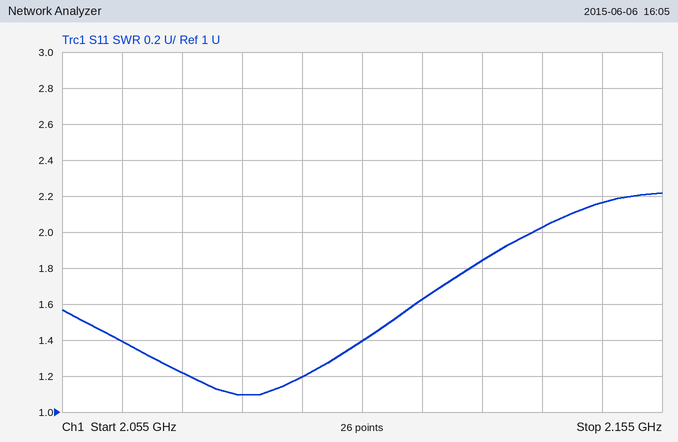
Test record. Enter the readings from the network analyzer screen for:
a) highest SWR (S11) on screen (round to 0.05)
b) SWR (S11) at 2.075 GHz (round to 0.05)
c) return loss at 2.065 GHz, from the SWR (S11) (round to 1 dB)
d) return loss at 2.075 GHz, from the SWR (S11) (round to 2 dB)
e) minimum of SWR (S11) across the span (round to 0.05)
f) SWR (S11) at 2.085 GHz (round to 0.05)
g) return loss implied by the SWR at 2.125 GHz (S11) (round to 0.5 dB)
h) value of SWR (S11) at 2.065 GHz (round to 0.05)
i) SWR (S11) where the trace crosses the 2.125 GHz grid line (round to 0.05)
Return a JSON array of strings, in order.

["2.20", "1.20", "16 dB", "20 dB", "1.10", "1.10", "10.5 dB", "1.40", "1.85"]
